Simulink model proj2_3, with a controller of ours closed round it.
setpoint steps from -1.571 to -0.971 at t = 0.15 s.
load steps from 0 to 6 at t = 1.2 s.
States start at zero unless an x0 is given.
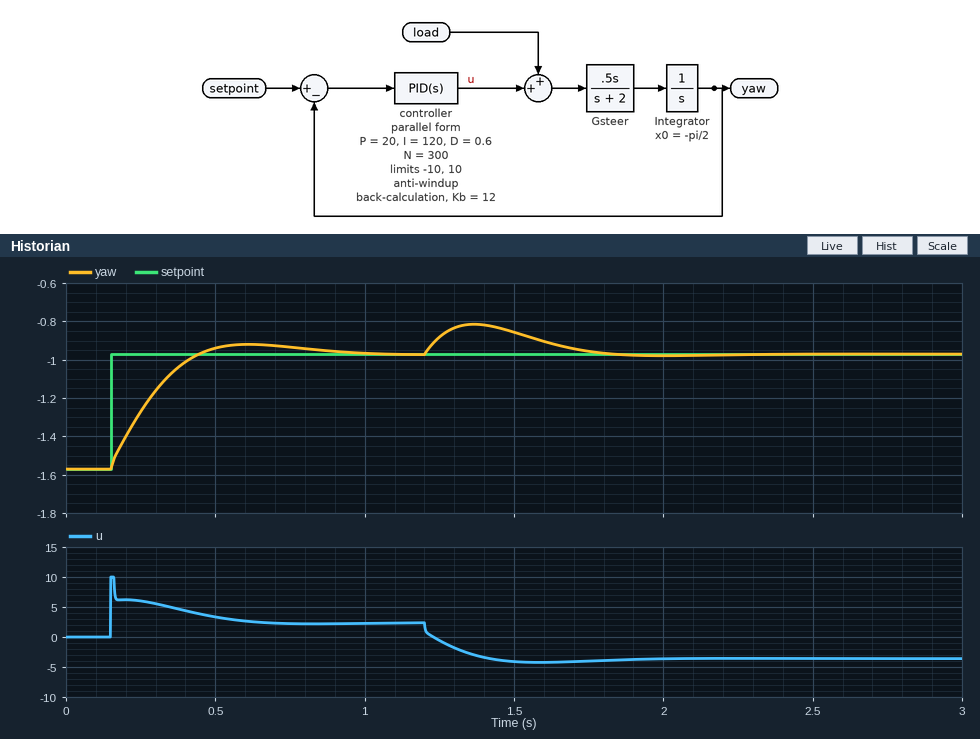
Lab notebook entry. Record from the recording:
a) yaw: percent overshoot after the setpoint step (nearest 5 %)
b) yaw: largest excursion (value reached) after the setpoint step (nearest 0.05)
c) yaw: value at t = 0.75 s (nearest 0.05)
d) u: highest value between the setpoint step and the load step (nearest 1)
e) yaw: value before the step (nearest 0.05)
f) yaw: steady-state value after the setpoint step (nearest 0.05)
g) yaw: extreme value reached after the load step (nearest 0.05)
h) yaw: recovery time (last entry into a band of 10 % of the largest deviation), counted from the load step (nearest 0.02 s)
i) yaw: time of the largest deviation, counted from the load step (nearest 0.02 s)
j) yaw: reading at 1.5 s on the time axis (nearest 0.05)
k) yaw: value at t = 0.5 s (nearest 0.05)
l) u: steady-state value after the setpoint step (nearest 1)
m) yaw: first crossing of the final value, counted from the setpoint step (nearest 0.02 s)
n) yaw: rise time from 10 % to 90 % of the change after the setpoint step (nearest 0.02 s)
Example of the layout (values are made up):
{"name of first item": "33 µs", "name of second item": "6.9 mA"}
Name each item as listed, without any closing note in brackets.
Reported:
{"yaw: percent overshoot after the setpoint step": "10 %", "yaw: largest excursion (value reached) after the setpoint step": "-0.90", "yaw: value at t = 0.75 s": "-0.95", "u: highest value between the setpoint step and the load step": "10", "yaw: value before the step": "-1.55", "yaw: steady-state value after the setpoint step": "-0.95", "yaw: extreme value reached after the load step": "-0.80", "yaw: recovery time (last entry into a band of 10 % of the largest deviation), counted from the load step": "0.54 s", "yaw: time of the largest deviation, counted from the load step": "0.16 s", "yaw: reading at 1.5 s on the time axis": "-0.85", "yaw: value at t = 0.5 s": "-0.95", "u: steady-state value after the setpoint step": "2", "yaw: first crossing of the final value, counted from the setpoint step": "0.30 s", "yaw: rise time from 10 % to 90 % of the change after the setpoint step": "0.22 s"}
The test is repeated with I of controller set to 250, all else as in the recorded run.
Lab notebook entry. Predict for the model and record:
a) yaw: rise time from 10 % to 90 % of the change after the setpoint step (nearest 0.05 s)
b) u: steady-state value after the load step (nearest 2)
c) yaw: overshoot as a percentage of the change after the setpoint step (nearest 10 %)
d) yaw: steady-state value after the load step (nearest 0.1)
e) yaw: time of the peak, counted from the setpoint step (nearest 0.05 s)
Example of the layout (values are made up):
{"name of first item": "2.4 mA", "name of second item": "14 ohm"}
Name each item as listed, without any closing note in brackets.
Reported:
{"yaw: rise time from 10 % to 90 % of the change after the setpoint step": "0.15 s", "u: steady-state value after the load step": "-4", "yaw: overshoot as a percentage of the change after the setpoint step": "20 %", "yaw: steady-state value after the load step": "-1.0", "yaw: time of the peak, counted from the setpoint step": "0.30 s"}
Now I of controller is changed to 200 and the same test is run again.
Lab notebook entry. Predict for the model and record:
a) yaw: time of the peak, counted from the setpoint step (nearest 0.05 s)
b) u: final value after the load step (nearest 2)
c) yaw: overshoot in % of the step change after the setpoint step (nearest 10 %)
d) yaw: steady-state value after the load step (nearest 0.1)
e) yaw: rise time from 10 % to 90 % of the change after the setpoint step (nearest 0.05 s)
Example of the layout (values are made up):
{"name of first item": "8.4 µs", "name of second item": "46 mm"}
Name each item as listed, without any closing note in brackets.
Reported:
{"yaw: time of the peak, counted from the setpoint step": "0.35 s", "u: final value after the load step": "-4", "yaw: overshoot in % of the step change after the setpoint step": "20 %", "yaw: steady-state value after the load step": "-1.0", "yaw: rise time from 10 % to 90 % of the change after the setpoint step": "0.15 s"}
